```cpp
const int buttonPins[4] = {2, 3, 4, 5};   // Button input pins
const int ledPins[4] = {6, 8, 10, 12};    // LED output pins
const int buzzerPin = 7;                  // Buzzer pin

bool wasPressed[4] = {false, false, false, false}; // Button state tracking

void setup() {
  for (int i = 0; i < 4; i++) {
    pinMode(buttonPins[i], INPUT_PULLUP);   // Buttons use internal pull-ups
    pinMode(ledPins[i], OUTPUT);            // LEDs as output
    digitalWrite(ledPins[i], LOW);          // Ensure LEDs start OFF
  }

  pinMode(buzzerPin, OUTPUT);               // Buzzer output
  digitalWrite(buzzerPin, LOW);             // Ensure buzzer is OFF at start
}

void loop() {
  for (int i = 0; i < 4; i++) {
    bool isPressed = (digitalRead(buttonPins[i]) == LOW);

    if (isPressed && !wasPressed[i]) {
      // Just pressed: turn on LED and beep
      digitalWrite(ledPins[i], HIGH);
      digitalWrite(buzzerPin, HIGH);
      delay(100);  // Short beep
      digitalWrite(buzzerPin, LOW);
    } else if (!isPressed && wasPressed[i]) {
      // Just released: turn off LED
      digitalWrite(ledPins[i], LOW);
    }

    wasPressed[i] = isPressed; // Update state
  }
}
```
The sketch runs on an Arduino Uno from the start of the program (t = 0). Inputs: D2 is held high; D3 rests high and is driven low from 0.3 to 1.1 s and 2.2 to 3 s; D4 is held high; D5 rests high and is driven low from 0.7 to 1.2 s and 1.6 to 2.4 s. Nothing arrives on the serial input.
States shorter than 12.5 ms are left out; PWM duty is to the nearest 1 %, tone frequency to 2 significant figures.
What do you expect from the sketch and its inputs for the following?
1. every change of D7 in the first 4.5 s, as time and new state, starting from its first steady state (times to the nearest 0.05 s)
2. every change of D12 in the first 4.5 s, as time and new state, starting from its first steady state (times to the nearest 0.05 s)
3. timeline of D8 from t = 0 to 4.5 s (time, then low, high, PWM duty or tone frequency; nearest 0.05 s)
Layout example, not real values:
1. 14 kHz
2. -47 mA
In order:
1. 0 s low; 0.3 s high; 0.4 s low; 0.7 s high; 0.8 s low; 1.6 s high; 1.7 s low; 2.2 s high; 2.3 s low
2. 0 s low; 0.7 s high; 1.2 s low; 1.6 s high; 2.4 s low
3. 0 s low; 0.3 s high; 1.1 s low; 2.2 s high; 3 s low
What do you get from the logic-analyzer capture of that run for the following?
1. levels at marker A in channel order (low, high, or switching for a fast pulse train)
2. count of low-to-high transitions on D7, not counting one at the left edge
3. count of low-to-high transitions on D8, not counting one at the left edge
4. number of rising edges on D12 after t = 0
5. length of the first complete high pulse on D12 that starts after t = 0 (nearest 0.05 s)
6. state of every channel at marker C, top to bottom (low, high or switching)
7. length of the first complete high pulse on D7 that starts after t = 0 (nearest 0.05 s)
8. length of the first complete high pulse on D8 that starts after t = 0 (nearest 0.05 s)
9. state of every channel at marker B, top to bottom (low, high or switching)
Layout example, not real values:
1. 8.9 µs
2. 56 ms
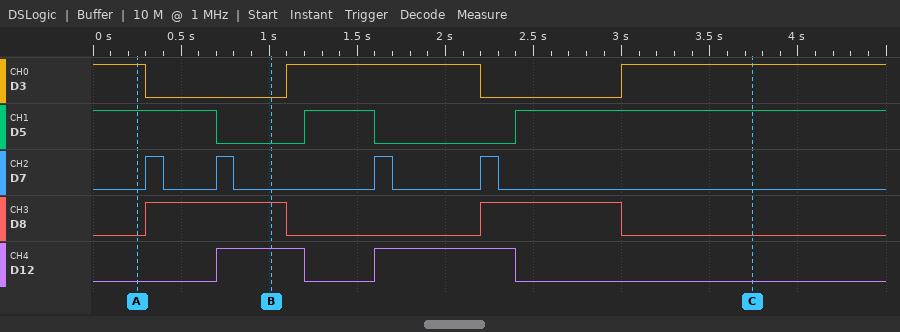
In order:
1. D3 high, D5 high, D7 low, D8 low, D12 low
2. 4
3. 2
4. 2
5. 0.50 s
6. D3 high, D5 high, D7 low, D8 low, D12 low
7. 0.10 s
8. 0.80 s
9. D3 low, D5 low, D7 low, D8 high, D12 high
